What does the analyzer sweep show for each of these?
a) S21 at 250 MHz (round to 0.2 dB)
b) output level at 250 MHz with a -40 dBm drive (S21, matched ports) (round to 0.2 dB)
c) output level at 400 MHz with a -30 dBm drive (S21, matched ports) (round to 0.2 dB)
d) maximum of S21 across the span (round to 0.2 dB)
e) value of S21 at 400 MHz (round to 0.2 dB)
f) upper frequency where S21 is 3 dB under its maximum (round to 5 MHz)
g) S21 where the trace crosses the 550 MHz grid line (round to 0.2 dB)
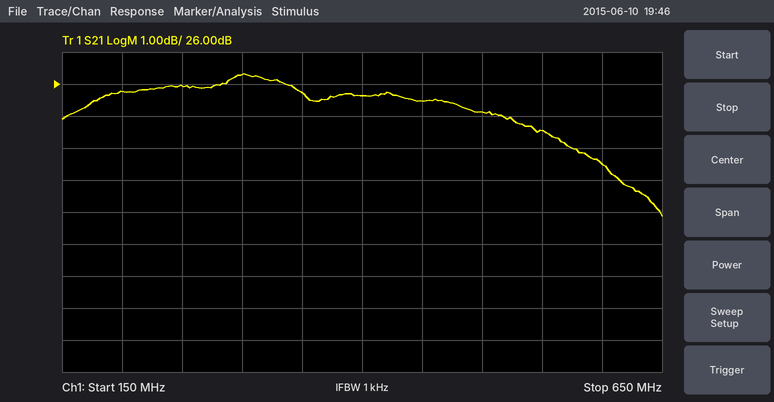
26.0 dB
-14.0 dBm
-4.4 dBm
26.4 dB
25.6 dB
605 MHz
24.6 dB
